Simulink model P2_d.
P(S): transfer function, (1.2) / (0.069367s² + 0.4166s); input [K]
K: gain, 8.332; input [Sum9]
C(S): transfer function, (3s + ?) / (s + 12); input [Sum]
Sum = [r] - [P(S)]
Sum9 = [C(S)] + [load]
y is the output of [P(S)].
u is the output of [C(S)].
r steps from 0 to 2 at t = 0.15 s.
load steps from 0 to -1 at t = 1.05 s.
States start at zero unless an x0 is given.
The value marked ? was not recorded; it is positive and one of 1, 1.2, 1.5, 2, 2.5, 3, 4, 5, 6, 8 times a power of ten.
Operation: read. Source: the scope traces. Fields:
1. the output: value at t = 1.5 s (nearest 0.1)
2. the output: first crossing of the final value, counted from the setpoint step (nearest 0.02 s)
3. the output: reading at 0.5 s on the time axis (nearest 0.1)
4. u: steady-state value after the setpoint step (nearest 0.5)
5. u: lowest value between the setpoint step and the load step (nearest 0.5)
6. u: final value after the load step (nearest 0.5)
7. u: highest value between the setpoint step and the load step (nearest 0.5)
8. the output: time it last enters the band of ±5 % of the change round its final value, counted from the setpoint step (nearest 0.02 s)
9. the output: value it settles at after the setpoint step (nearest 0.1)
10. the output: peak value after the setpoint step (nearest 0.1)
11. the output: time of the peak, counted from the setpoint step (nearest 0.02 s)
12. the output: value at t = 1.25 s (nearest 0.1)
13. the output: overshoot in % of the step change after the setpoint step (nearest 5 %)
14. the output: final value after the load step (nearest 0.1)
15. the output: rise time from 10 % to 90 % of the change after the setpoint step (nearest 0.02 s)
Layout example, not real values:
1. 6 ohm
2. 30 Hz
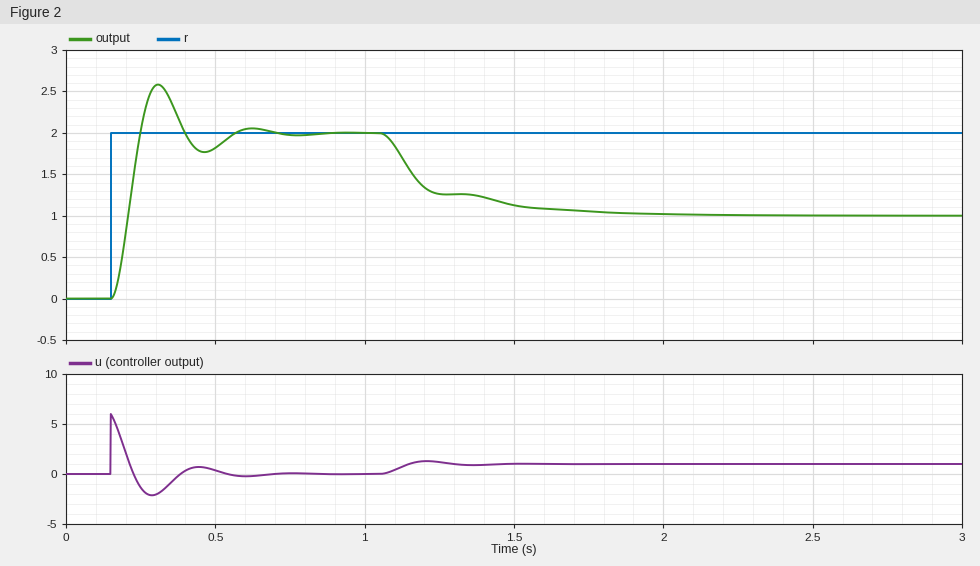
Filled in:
1. 1.1
2. 0.10 s
3. 1.8
4. 0.0
5. -2.0
6. 1.0
7. 6.0
8. 0.38 s
9. 2.0
10. 2.6
11. 0.16 s
12. 1.3
13. 30 %
14. 1.0
15. 0.06 s
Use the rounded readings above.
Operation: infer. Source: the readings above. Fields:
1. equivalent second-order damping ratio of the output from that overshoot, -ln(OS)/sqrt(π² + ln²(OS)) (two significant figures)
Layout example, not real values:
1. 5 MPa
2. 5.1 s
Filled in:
1. 0.36
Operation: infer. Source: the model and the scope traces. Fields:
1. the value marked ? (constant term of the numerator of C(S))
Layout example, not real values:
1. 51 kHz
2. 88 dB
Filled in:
1. 12
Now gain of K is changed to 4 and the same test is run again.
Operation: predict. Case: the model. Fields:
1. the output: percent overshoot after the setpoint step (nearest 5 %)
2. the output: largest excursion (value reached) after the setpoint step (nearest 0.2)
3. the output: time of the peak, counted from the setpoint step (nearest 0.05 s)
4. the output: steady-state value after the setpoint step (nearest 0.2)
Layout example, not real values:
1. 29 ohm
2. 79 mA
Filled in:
1. 10 %
2. 2.2
3. 0.25 s
4. 2.0
